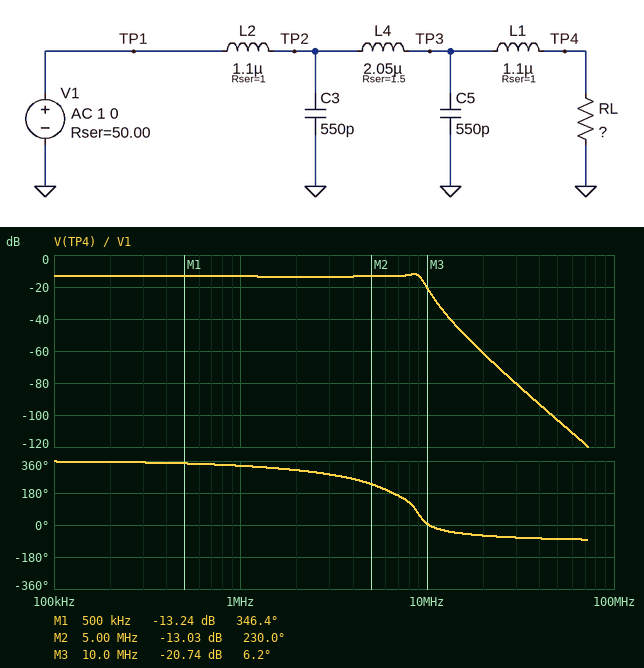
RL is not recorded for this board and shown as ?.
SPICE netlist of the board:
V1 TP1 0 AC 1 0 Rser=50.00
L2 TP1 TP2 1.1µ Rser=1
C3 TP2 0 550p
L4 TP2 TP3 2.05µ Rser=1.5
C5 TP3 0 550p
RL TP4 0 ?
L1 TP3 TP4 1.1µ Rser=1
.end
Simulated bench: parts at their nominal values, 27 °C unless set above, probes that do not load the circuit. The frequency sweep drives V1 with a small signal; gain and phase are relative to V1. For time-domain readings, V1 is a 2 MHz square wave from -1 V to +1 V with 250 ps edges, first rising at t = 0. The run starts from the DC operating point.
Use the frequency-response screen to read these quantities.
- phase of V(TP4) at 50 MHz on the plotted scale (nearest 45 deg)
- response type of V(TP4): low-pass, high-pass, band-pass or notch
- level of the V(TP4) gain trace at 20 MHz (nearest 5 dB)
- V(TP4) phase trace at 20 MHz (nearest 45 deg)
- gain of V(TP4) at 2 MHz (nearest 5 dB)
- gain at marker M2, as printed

-90 deg
low-pass
-60 dB
-45 deg
-15 dB
-13.03 dB
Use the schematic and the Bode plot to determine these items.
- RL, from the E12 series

15 Ω
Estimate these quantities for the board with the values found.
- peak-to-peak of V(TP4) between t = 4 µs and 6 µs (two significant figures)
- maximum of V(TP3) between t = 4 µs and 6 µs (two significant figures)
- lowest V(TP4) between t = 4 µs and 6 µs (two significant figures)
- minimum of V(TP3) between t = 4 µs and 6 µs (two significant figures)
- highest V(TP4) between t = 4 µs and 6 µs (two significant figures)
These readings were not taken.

560 mV
680 mV
-280 mV
-680 mV
280 mV
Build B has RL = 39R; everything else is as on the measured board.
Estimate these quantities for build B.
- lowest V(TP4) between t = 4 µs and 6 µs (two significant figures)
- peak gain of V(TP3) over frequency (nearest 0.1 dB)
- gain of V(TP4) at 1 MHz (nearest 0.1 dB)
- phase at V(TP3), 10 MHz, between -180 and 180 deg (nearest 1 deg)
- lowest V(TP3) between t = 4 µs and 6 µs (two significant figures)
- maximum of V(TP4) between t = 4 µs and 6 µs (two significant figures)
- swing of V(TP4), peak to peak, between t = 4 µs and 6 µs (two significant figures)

-540 mV
-2.9 dB
-7.6 dB
89 deg
-720 mV
540 mV
1.1 V
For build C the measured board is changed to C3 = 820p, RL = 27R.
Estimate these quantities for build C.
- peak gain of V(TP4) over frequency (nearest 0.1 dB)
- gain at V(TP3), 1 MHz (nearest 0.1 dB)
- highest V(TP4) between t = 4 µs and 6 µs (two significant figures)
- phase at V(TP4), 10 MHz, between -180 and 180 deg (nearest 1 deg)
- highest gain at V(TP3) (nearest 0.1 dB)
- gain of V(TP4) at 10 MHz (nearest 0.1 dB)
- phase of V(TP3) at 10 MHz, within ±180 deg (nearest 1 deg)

-9.5 dB
-8.9 dB
410 mV
4 deg
-4.3 dB
-23.4 dB
72 deg
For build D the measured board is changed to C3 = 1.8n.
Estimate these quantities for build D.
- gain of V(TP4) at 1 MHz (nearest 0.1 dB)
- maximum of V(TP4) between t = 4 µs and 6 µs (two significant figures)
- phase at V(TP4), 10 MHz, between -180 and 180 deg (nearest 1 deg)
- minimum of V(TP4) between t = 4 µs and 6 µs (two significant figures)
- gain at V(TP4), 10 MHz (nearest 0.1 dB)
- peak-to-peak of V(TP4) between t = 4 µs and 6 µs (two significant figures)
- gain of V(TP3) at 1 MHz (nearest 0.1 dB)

-12.8 dB
290 mV
-21 deg
-290 mV
-36.2 dB
580 mV
-11.5 dB
